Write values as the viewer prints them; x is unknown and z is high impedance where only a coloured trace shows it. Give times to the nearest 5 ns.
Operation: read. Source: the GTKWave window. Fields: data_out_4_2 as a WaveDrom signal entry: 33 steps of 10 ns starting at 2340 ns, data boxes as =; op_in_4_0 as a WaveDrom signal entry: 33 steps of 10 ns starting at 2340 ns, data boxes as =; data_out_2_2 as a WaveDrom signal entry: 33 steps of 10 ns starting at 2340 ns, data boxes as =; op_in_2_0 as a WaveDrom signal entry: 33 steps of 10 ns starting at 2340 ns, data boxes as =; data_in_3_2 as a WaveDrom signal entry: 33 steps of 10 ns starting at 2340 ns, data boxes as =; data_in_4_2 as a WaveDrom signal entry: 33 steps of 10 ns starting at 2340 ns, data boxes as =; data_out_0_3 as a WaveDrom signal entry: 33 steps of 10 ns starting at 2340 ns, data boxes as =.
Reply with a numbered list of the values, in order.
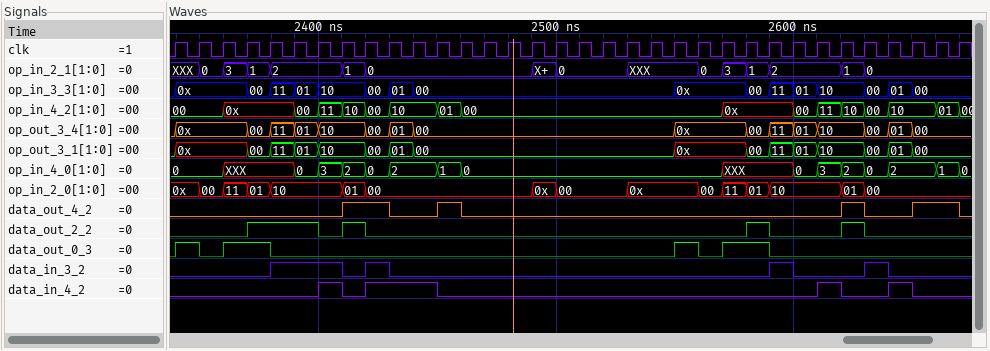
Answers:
1. {name: 'data_out_4_2', wave: '0......1.0.10...............10.1.'}
2. {name: 'op_in_4_0', wave: '=.=..=====.==..........=..=====.=', data: '0 XXX 0 3 2 0 2 1 0 XXX 0 3 2 0 2 1'}
3. {name: 'data_out_2_2', wave: '0..1..010...............10..10...'}
4. {name: 'op_in_2_0', wave: '=====..==......==..=..====..==...', data: '0x 00 11 01 10 01 00 0x 00 0x 00 11 01 10 01 00'}
5. {name: 'data_in_3_2', wave: '0...1..010...............10..10..'}
6. {name: 'data_in_4_2', wave: '0.....101..0...............10.10.'}
7. {name: 'data_out_0_3', wave: '101.0................101.0.......'}
